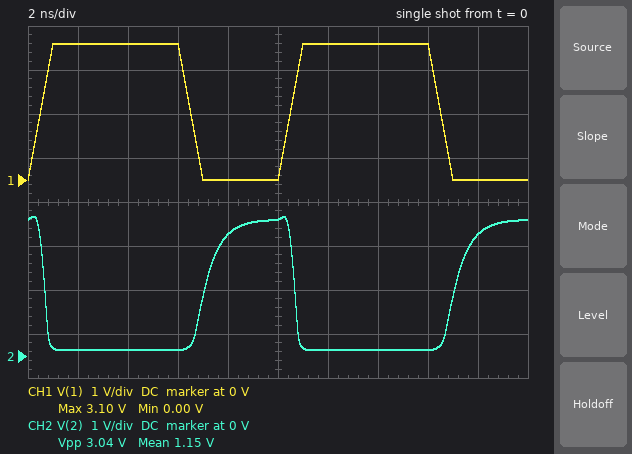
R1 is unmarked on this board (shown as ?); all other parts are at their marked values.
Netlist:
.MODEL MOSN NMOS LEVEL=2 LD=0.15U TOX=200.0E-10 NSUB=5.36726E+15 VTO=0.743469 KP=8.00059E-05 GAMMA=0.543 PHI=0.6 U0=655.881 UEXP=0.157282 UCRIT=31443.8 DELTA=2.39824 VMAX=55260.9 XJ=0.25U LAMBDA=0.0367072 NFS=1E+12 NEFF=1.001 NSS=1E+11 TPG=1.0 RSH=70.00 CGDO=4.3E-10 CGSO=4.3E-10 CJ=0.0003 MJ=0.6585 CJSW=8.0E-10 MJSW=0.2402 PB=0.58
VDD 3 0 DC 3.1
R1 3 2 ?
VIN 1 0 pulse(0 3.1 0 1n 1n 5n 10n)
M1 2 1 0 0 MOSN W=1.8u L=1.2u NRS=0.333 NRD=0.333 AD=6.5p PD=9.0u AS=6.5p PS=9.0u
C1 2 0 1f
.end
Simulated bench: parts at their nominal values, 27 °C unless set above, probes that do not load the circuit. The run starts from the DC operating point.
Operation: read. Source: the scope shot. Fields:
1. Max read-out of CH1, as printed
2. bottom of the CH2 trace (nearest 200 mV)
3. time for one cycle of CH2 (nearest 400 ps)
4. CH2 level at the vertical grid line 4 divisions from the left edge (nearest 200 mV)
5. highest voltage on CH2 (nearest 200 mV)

3.10 V
200 mV
10.0 ns
2.8 V
3.2 V
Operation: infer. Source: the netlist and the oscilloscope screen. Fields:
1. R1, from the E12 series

82 kΩ
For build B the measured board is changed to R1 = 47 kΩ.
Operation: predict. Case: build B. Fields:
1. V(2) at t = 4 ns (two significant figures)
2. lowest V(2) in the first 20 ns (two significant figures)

250 mV
240 mV
